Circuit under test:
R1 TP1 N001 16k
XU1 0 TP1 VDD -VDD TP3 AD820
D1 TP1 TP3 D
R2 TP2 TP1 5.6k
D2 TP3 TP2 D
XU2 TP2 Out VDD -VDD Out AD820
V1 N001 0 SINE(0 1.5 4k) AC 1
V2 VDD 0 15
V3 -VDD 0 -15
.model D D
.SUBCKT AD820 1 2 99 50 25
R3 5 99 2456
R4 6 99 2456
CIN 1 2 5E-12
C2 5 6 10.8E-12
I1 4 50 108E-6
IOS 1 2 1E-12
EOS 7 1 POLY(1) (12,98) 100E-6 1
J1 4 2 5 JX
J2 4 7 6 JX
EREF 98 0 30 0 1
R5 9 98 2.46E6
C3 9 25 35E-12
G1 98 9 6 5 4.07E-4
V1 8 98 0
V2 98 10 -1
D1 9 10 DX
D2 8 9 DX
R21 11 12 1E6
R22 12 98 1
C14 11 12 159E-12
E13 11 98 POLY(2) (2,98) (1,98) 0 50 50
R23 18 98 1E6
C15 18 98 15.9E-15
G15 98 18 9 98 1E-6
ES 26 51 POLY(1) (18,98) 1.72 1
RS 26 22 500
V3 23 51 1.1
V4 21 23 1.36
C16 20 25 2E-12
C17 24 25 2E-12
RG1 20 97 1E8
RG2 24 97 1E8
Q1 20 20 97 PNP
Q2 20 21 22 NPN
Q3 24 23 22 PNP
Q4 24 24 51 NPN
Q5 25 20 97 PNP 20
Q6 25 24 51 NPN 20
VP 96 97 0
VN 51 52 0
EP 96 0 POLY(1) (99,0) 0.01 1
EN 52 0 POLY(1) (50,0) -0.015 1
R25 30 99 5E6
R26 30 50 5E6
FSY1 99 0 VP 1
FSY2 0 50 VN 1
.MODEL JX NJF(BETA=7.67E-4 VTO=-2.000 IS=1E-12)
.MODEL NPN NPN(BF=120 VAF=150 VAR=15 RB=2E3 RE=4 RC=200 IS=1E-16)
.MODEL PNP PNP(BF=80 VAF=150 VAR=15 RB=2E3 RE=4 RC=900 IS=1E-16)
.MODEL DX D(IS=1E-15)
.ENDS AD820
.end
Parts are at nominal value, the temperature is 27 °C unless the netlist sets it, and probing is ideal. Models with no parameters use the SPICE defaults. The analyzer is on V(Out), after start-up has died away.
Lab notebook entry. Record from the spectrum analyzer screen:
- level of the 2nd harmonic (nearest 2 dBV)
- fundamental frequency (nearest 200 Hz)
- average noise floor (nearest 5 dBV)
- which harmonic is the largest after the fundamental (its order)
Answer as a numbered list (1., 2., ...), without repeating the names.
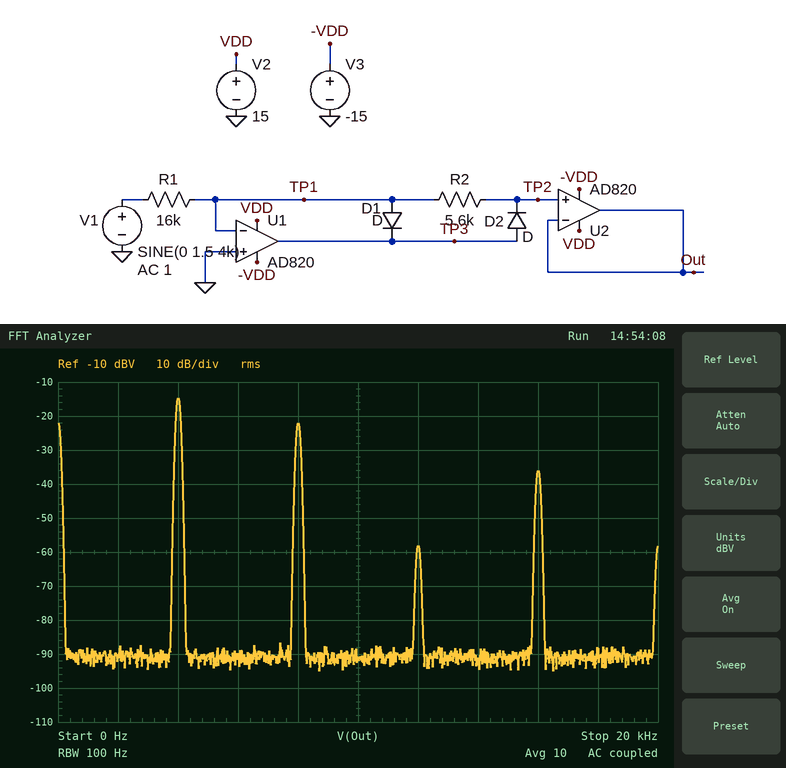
1. -22 dBV
2. 4.0 kHz
3. -90 dBV
4. 2
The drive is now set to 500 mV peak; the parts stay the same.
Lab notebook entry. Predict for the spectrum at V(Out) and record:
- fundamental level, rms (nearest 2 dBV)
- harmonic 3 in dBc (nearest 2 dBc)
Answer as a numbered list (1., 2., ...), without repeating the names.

1. -24 dBV
2. -34 dBc
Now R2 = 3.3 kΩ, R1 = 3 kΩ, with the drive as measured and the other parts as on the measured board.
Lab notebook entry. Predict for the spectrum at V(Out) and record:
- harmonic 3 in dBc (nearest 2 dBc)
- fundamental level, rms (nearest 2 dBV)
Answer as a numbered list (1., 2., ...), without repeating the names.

1. -50 dBc
2. -4 dBV
